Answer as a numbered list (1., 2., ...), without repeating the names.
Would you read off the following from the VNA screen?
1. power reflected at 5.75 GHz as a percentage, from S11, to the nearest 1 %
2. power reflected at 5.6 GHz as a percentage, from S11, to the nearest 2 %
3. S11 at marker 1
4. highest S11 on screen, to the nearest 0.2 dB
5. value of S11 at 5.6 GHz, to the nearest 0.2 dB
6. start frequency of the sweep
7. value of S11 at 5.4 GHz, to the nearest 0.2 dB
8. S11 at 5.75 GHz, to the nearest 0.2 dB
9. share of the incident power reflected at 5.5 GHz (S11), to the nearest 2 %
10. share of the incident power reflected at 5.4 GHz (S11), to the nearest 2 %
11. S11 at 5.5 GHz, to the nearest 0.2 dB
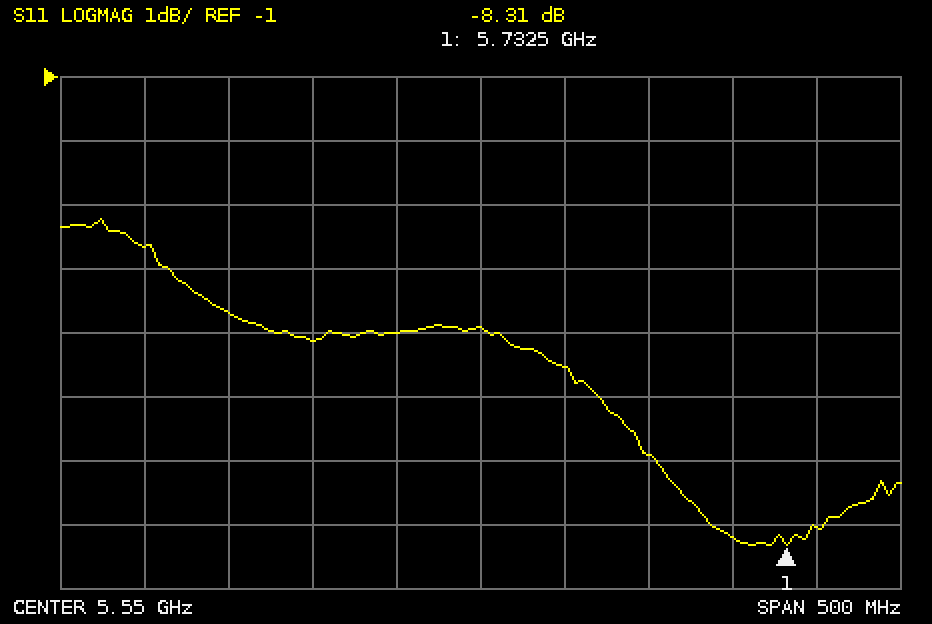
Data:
1. 16 %
2. 28 %
3. -8.31 dB
4. -3.2 dB
5. -5.6 dB
6. 5.3 GHz
7. -4.6 dB
8. -8.0 dB
9. 32 %
10. 34 %
11. -5.0 dB
